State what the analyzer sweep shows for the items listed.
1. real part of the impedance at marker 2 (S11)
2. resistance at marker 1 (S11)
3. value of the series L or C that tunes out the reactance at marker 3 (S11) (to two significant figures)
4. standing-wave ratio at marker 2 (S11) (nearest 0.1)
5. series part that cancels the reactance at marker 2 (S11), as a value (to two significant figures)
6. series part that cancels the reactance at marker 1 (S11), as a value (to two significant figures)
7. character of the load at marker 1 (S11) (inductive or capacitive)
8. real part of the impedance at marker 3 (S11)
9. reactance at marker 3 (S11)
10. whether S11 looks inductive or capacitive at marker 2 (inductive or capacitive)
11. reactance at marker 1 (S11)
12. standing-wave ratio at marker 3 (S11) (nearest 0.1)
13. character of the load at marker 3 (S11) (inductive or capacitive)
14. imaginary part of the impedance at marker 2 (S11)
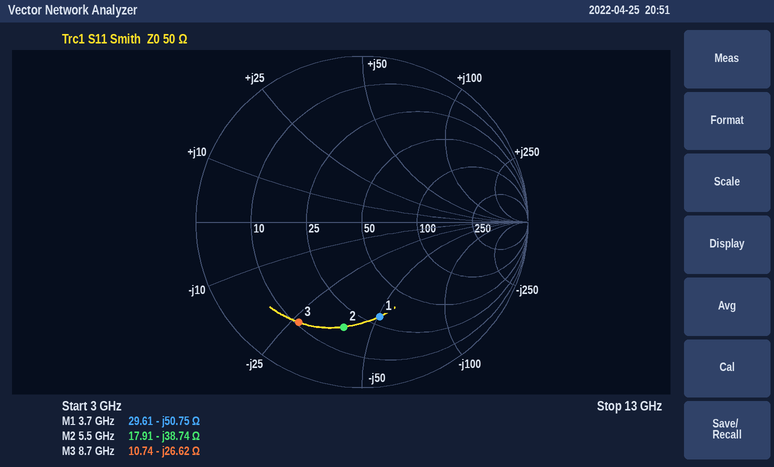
17.91 Ω
29.61 Ω
490 pH
4.6
1.1 nH
2.2 nH
capacitive
10.74 Ω
-26.62 Ω
capacitive
-50.75 Ω
6.0
capacitive
-38.74 Ω
